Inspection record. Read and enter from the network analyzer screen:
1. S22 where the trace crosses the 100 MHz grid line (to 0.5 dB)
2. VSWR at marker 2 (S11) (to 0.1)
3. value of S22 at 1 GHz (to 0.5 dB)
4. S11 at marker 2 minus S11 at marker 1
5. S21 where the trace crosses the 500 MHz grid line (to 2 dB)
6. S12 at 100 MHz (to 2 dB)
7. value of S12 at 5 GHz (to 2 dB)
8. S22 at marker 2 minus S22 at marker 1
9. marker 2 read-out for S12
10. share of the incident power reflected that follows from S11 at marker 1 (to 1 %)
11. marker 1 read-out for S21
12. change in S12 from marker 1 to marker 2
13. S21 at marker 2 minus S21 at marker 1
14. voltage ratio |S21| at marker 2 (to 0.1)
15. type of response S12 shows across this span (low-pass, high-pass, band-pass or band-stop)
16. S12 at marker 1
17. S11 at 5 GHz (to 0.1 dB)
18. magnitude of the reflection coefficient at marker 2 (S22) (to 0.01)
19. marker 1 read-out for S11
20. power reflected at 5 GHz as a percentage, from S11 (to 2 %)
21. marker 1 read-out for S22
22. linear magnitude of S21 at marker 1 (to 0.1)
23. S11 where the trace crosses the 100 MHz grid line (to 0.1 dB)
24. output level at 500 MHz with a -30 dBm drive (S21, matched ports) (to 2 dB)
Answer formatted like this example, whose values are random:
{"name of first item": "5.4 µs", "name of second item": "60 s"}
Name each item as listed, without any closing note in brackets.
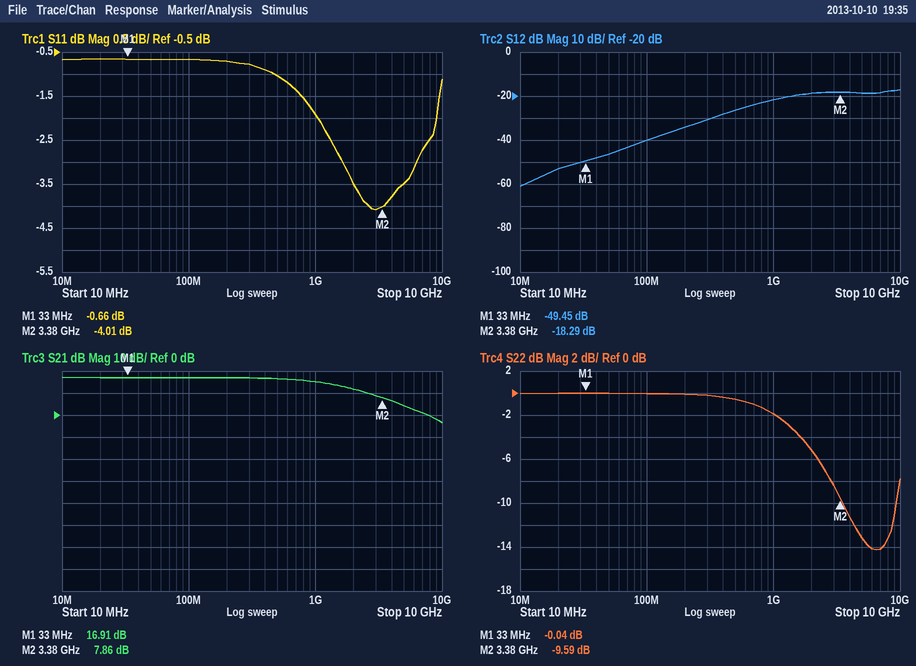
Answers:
{"S22 where the trace crosses the 100 MHz grid line": "0.0 dB", "VSWR at marker 2 (S11)": "4.4", "value of S22 at 1 GHz": "-2.0 dB", "S11 at marker 2 minus S11 at marker 1": "-3.35 dB", "S21 where the trace crosses the 500 MHz grid line": "16 dB", "S12 at 100 MHz": "-40 dB", "value of S12 at 5 GHz": "-18 dB", "S22 at marker 2 minus S22 at marker 1": "-9.55 dB", "marker 2 read-out for S12": "-18.29 dB", "share of the incident power reflected that follows from S11 at marker 1": "86 %", "marker 1 read-out for S21": "16.91 dB", "change in S12 from marker 1 to marker 2": "31.16 dB", "S21 at marker 2 minus S21 at marker 1": "-9.05 dB", "voltage ratio |S21| at marker 2": "2.5", "type of response S12 shows across this span": "high-pass", "S12 at marker 1": "-49.45 dB", "S11 at 5 GHz": "-3.5 dB", "magnitude of the reflection coefficient at marker 2 (S22)": "0.33", "marker 1 read-out for S11": "-0.66 dB", "power reflected at 5 GHz as a percentage, from S11": "44 %", "marker 1 read-out for S22": "-0.04 dB", "linear magnitude of S21 at marker 1": "7.0", "S11 where the trace crosses the 100 MHz grid line": "-0.7 dB", "output level at 500 MHz with a -30 dBm drive (S21, matched ports)": "-14 dBm"}
